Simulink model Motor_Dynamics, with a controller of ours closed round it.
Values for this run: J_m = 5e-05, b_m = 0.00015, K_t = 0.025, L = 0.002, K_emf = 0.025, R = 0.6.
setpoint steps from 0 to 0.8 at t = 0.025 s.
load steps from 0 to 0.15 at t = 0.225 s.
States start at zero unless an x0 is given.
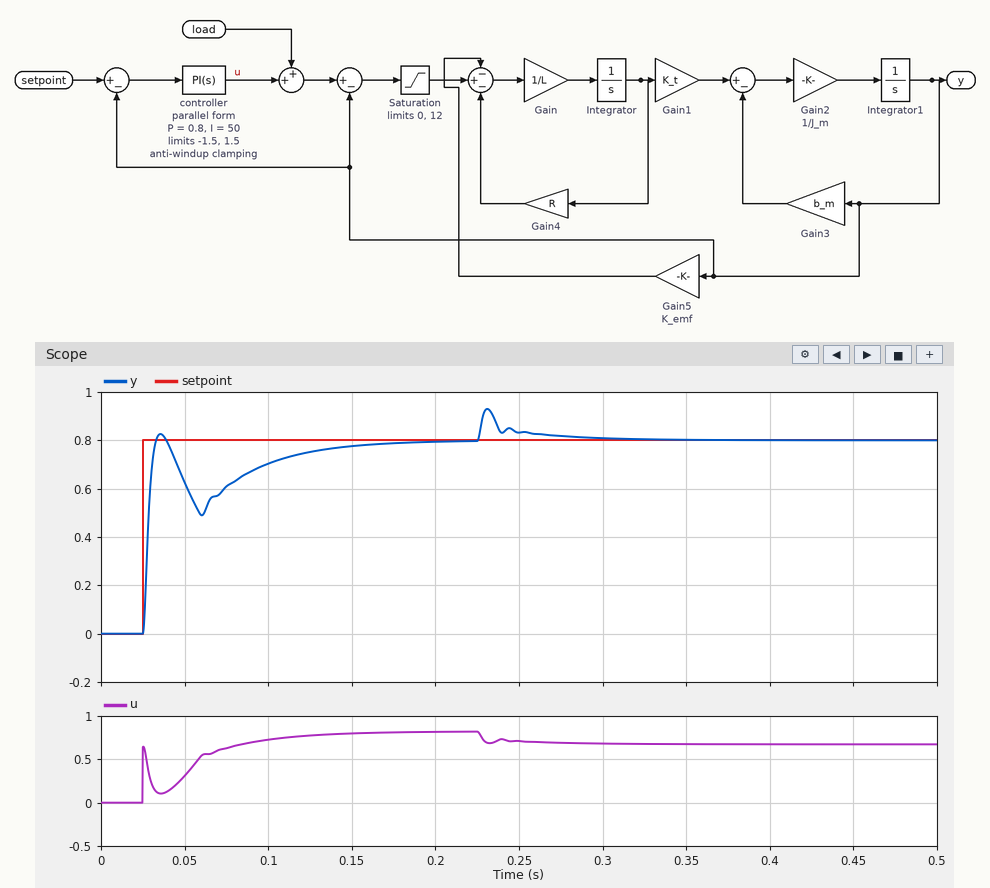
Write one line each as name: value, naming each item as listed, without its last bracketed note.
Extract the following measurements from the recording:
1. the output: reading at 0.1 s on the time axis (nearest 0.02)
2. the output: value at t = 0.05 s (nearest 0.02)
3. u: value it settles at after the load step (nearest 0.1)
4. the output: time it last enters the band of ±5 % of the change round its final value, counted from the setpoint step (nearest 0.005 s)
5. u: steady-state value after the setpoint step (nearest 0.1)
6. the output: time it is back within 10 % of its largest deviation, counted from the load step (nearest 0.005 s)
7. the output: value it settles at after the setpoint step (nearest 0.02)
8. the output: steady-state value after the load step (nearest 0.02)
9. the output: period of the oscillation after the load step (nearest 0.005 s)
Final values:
the output: reading at 0.1 s on the time axis: 0.70
the output: value at t = 0.05 s: 0.62
u: value it settles at after the load step: 0.7
the output: time it last enters the band of ±5 % of the change round its final value, counted from the setpoint step: 0.105 s
u: steady-state value after the setpoint step: 0.8
the output: time it is back within 10 % of its largest deviation, counted from the load step: 0.060 s
the output: value it settles at after the setpoint step: 0.80
the output: steady-state value after the load step: 0.80
the output: period of the oscillation after the load step: 0.015 s
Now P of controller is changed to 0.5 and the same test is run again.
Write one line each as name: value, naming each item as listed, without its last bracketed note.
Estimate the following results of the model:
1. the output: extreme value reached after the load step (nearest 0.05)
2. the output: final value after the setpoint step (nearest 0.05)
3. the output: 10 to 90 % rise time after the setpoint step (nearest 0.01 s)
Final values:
the output: extreme value reached after the load step: 0.95
the output: final value after the setpoint step: 0.80
the output: 10 to 90 % rise time after the setpoint step: 0.06 s
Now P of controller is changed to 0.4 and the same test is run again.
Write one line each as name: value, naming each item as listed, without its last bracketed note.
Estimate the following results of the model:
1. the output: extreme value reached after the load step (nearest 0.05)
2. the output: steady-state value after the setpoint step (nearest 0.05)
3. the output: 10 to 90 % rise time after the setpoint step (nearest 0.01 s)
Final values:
the output: extreme value reached after the load step: 0.95
the output: steady-state value after the setpoint step: 0.80
the output: 10 to 90 % rise time after the setpoint step: 0.06 s
